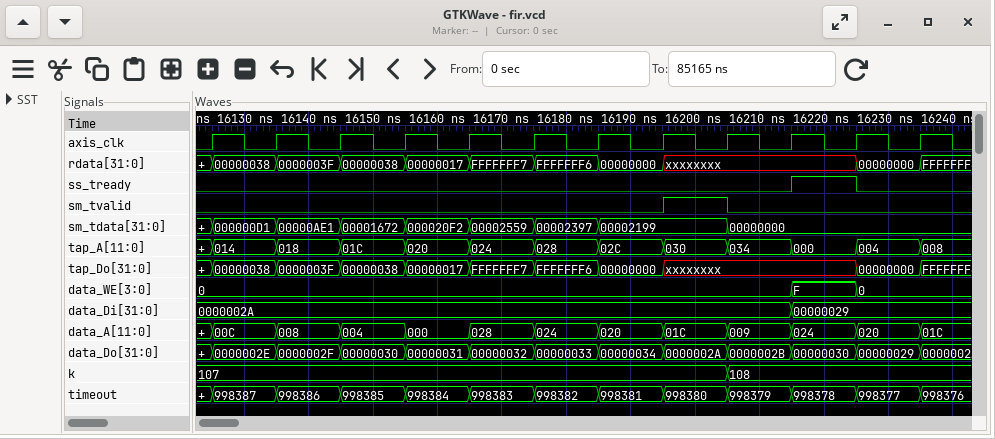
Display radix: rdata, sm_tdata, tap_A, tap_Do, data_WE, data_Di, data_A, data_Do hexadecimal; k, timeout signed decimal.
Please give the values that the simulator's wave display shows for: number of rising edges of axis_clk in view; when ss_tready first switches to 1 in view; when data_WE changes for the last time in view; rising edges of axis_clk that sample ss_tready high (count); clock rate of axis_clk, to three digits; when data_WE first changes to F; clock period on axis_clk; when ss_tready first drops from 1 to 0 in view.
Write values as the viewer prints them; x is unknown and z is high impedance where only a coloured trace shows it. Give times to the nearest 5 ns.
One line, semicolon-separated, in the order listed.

12; 16215 ns; 16225 ns; 1; 100 MHz; 16215 ns; 10 ns; 16225 ns
